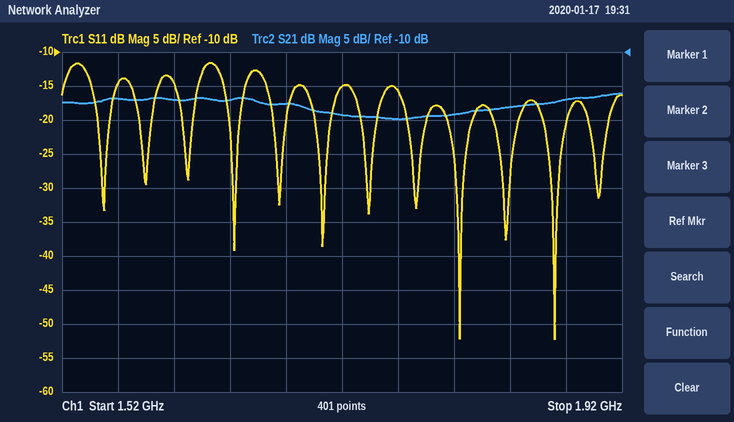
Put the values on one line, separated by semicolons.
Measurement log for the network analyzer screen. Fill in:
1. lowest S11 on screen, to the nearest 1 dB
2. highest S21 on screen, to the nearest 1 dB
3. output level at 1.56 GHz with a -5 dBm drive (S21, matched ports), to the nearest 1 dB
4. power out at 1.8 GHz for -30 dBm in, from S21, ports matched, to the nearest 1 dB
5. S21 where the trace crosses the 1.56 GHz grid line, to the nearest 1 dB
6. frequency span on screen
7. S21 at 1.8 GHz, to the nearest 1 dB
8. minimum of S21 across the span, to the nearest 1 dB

-52 dB; -16 dB; -22 dBm; -49 dBm; -17 dB; 400 MHz; -19 dB; -20 dB
